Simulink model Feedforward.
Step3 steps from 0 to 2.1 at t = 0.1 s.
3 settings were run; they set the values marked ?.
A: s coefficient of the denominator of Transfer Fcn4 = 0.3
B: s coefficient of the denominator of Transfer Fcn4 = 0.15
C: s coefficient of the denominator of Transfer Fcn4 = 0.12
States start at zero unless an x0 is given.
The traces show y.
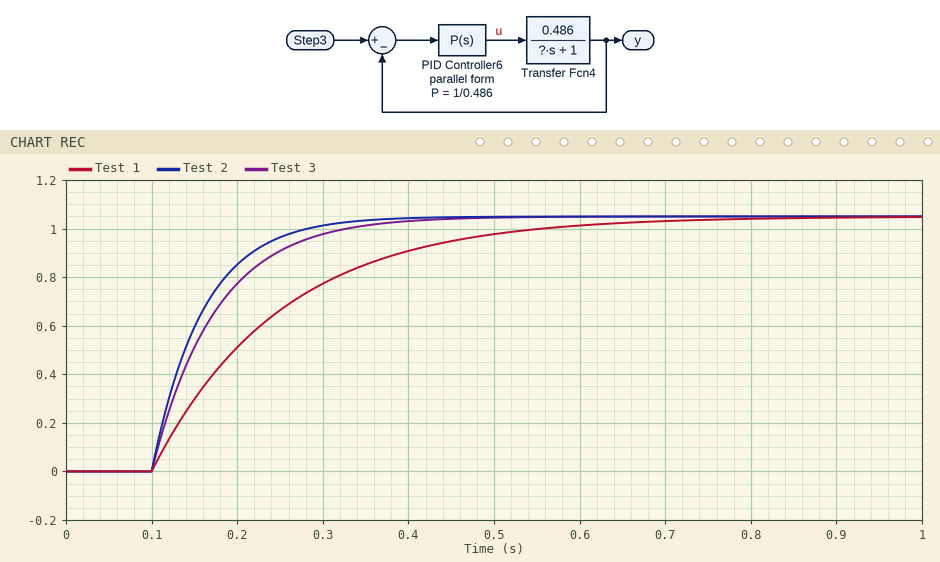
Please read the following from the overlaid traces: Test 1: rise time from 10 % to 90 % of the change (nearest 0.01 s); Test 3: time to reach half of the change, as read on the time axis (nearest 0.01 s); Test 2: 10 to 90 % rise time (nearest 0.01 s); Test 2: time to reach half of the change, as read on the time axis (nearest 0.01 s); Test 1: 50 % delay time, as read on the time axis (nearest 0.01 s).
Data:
0.33 s
0.15 s
0.13 s
0.14 s
0.20 s
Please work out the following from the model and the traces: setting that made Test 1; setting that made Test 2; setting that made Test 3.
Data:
A
C
B
